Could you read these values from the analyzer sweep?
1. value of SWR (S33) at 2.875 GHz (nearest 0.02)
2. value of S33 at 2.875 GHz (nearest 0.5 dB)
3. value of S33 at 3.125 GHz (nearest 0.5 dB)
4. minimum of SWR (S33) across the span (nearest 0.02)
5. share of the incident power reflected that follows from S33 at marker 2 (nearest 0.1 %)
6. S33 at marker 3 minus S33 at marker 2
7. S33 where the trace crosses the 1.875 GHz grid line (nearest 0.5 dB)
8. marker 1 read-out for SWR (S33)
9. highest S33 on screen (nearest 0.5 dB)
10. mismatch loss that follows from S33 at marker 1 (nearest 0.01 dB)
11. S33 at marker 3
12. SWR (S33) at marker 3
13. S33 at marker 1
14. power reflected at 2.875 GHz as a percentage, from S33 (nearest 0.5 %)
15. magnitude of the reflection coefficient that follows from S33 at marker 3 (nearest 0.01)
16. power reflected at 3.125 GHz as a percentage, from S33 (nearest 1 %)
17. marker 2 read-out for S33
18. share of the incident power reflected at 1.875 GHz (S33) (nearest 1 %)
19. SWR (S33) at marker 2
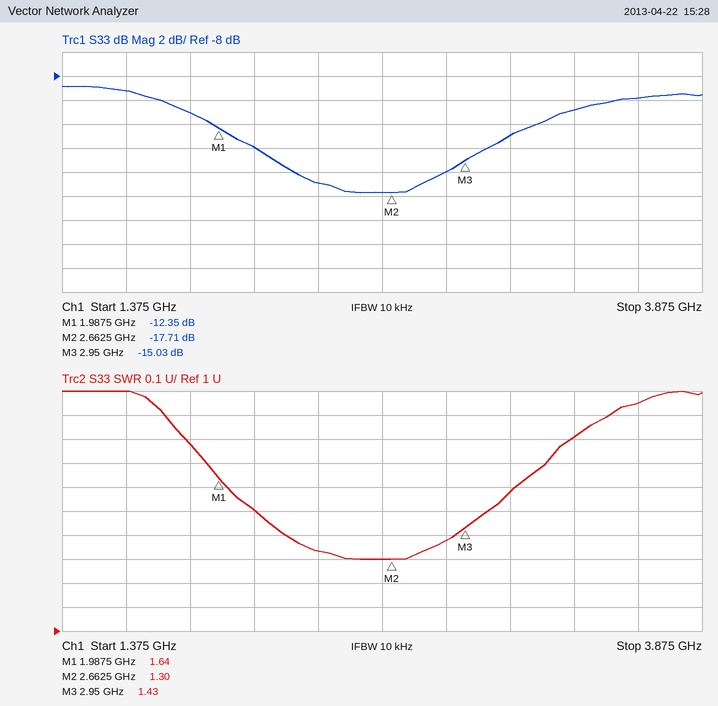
1.38
-16.0 dB
-13.0 dB
1.30
1.7 %
2.68 dB
-11.0 dB
1.64
-9.0 dB
0.26 dB
-15.03 dB
1.43
-12.35 dB
2.5 %
0.18
5 %
-17.71 dB
8 %
1.30
